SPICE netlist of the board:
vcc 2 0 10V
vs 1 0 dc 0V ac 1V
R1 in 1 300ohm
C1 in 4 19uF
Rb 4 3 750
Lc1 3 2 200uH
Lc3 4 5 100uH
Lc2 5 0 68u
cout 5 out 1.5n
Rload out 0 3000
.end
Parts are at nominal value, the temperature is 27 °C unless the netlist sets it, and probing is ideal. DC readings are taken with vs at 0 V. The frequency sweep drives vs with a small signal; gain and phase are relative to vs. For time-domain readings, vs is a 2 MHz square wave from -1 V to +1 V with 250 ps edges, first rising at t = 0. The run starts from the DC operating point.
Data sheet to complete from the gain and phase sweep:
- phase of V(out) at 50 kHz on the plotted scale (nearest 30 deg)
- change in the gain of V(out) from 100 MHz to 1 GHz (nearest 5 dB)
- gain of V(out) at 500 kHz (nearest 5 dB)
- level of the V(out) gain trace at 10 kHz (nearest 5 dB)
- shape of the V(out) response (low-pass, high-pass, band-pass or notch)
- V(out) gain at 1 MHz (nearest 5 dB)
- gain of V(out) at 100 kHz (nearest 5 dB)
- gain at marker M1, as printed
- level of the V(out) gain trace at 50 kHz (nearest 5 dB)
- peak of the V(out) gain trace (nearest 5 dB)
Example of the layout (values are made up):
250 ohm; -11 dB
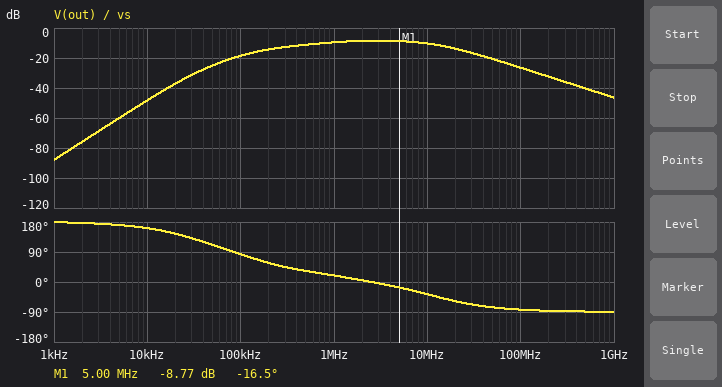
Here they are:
120 deg; -20 dB; -10 dB; -50 dB; band-pass; -10 dB; -20 dB; -8.77 dB; -25 dB; -10 dB
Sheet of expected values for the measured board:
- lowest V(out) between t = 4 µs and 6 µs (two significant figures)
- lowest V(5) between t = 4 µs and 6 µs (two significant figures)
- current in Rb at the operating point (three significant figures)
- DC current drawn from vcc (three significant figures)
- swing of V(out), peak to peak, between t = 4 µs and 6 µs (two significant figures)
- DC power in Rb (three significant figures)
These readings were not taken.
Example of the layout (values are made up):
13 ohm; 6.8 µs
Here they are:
-480 mV; -460 mV; 13.3 mA; 13.3 mA; 930 mV; 133 mW
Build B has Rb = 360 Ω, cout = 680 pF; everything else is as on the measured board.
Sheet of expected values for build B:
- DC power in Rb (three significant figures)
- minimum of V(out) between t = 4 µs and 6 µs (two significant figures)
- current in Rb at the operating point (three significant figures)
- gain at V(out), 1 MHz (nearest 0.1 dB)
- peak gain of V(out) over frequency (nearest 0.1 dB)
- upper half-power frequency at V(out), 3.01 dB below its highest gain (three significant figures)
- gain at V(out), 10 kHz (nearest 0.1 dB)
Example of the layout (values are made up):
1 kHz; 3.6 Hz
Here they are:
278 mW; -500 mV; 27.8 mA; -9.4 dB; -8.4 dB; 13.1 MHz; -54.9 dB
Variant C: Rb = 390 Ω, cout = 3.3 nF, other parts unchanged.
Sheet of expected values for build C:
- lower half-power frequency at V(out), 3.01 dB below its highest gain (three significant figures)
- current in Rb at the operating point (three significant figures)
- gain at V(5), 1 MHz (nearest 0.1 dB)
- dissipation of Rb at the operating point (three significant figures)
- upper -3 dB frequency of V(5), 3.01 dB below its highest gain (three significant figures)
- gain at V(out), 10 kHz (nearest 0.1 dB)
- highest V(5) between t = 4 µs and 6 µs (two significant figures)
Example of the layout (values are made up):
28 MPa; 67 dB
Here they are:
515 kHz; 25.6 mA; -9.4 dB; 256 mW; 13.2 MHz; -42.5 dB; 470 mV
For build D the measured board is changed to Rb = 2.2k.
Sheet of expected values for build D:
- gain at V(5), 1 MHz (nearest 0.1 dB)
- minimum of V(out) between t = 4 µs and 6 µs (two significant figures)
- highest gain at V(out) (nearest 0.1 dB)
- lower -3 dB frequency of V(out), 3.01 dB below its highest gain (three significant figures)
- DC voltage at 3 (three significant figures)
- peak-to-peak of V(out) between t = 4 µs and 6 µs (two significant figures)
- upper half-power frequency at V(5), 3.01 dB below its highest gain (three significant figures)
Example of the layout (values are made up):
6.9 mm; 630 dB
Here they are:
-9.2 dB; -460 mV; -8.6 dB; 284 kHz; 10.0 V; 890 mV; 13.7 MHz
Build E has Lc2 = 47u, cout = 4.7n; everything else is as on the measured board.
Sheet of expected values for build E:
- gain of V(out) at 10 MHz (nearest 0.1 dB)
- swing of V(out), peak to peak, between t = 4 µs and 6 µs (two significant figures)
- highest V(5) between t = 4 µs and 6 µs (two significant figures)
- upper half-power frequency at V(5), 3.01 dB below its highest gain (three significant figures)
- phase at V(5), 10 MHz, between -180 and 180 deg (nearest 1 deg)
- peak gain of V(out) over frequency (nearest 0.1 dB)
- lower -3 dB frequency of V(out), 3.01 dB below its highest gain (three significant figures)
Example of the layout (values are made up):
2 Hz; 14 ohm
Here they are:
-11.6 dB; 760 mV; 380 mV; 16.5 MHz; -30 deg; -10.4 dB; 506 kHz
